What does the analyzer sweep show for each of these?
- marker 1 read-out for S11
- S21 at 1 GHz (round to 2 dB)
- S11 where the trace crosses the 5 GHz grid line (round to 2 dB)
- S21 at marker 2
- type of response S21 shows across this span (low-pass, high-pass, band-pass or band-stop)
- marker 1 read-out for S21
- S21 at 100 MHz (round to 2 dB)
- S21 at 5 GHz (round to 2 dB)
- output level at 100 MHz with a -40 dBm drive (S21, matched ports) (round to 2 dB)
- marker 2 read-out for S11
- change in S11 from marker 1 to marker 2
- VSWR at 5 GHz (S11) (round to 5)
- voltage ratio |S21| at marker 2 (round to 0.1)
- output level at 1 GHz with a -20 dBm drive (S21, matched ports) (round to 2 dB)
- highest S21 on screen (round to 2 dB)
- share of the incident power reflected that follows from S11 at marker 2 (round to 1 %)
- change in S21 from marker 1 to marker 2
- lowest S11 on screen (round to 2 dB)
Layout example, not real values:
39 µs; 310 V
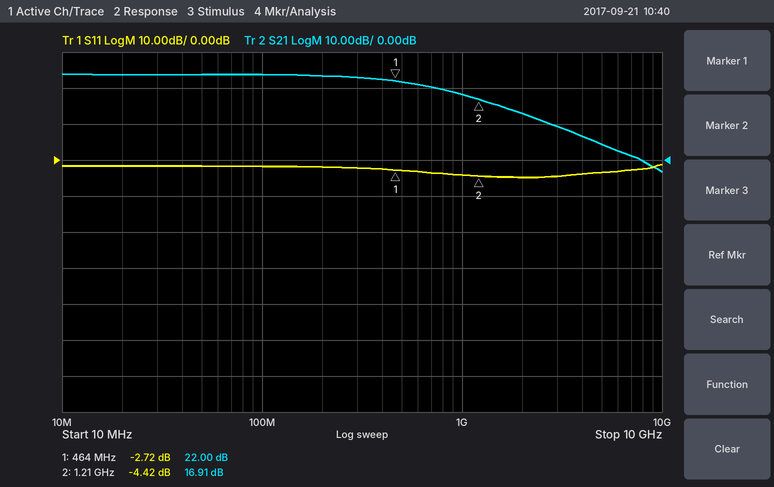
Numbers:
-2.72 dB; 18 dB; -4 dB; 16.91 dB; low-pass; 22.00 dB; 24 dB; 4 dB; -16 dBm; -4.42 dB; -1.70 dB; 5; 7.0; -2 dBm; 24 dB; 36 %; -5.09 dB; -4 dB
